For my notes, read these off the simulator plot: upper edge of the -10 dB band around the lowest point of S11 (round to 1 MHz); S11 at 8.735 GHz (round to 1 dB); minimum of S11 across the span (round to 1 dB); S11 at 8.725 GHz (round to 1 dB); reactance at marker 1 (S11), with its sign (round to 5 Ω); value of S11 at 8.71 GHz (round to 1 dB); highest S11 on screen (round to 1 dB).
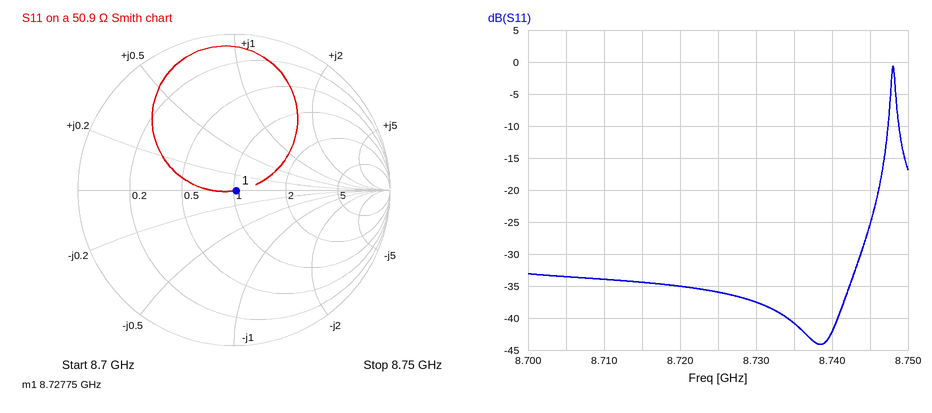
8.747 GHz
-41 dB
-44 dB
-36 dB
0 Ω
-34 dB
-1 dB
